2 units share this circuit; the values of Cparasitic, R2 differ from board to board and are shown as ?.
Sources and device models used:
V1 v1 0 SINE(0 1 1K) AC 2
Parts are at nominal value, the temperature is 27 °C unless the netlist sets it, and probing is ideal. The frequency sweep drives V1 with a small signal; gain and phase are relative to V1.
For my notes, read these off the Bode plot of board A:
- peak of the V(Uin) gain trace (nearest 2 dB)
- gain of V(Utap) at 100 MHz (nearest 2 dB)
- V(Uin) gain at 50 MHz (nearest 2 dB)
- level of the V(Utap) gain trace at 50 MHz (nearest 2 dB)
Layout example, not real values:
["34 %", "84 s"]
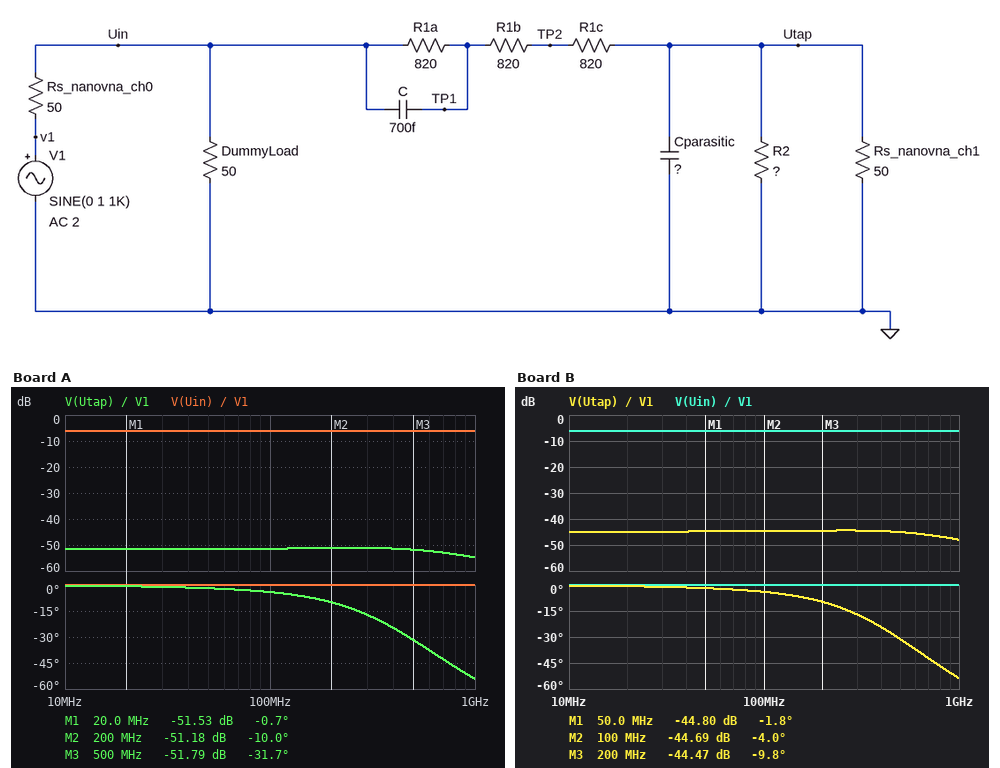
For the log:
["-6 dB", "-52 dB", "-6 dB", "-52 dB"]
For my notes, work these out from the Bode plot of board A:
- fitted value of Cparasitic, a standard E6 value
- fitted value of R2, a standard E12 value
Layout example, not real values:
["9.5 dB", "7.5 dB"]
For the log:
["22 pF", "18 Ω"]
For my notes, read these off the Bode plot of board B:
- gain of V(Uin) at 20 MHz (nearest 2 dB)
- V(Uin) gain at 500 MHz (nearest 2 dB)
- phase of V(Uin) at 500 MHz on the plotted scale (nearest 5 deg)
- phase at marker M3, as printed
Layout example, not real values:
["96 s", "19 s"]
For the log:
["-6 dB", "-6 dB", "0 deg", "-9.8 deg"]
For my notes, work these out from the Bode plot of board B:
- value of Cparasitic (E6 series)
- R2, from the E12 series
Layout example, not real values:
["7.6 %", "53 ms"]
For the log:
["10 pF", "68 Ω"]
